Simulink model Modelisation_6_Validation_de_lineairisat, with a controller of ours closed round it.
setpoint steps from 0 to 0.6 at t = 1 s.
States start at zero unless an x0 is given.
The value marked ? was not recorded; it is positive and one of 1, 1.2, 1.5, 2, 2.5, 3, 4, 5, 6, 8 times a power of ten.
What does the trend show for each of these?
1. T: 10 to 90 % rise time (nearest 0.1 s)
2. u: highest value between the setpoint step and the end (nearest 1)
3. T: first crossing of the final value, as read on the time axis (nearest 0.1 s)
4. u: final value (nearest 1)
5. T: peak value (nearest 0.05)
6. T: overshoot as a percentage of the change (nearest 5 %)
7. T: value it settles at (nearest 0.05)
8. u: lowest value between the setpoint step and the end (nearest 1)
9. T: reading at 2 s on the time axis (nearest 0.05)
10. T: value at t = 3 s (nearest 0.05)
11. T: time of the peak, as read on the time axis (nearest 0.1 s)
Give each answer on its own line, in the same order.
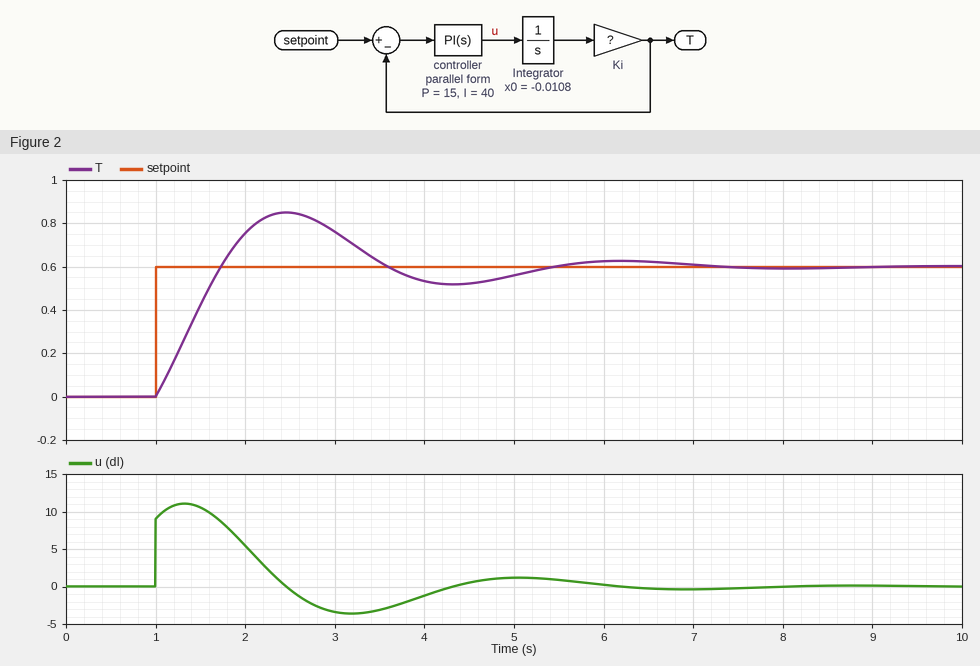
0.6 s
11
1.7 s
0
0.85
40 %
0.60
-4
0.75
0.75
2.5 s
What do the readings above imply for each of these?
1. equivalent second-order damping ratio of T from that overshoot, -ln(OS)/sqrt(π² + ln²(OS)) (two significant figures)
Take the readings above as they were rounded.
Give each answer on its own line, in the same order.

0.28
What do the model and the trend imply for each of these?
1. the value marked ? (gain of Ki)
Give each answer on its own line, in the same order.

0.08
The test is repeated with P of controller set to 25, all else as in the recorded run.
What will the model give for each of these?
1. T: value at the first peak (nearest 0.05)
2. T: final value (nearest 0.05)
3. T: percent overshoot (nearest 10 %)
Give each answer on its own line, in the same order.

0.75
0.60
30 %
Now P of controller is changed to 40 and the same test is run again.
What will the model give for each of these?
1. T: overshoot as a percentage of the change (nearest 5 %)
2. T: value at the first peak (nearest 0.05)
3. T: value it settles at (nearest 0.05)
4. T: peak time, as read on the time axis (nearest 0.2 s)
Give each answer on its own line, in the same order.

15 %
0.70
0.60
2.2 s
